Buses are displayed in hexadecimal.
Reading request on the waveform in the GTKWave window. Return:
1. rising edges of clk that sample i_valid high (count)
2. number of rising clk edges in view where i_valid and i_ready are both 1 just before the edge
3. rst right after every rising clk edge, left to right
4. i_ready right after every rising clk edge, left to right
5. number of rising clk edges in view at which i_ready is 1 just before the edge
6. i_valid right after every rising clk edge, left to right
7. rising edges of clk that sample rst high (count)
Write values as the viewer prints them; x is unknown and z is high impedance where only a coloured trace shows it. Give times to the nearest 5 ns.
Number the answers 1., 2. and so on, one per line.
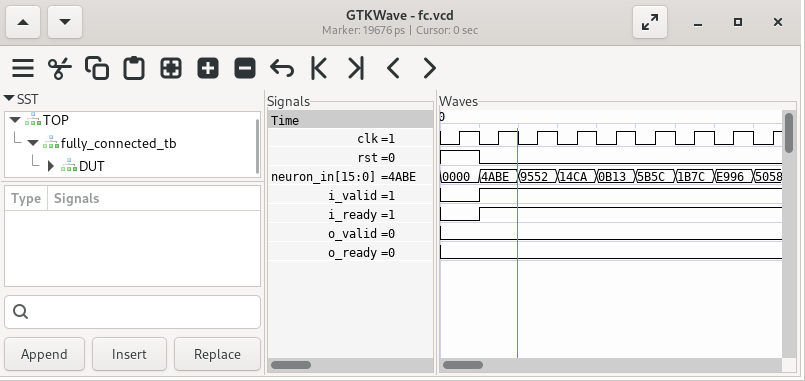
1. 8
2. 8
3. 1 0 0 0 0 0 0 0 0
4. 0 1 1 1 1 1 1 1 1
5. 8
6. 0 1 1 1 1 1 1 1 1
7. 1
